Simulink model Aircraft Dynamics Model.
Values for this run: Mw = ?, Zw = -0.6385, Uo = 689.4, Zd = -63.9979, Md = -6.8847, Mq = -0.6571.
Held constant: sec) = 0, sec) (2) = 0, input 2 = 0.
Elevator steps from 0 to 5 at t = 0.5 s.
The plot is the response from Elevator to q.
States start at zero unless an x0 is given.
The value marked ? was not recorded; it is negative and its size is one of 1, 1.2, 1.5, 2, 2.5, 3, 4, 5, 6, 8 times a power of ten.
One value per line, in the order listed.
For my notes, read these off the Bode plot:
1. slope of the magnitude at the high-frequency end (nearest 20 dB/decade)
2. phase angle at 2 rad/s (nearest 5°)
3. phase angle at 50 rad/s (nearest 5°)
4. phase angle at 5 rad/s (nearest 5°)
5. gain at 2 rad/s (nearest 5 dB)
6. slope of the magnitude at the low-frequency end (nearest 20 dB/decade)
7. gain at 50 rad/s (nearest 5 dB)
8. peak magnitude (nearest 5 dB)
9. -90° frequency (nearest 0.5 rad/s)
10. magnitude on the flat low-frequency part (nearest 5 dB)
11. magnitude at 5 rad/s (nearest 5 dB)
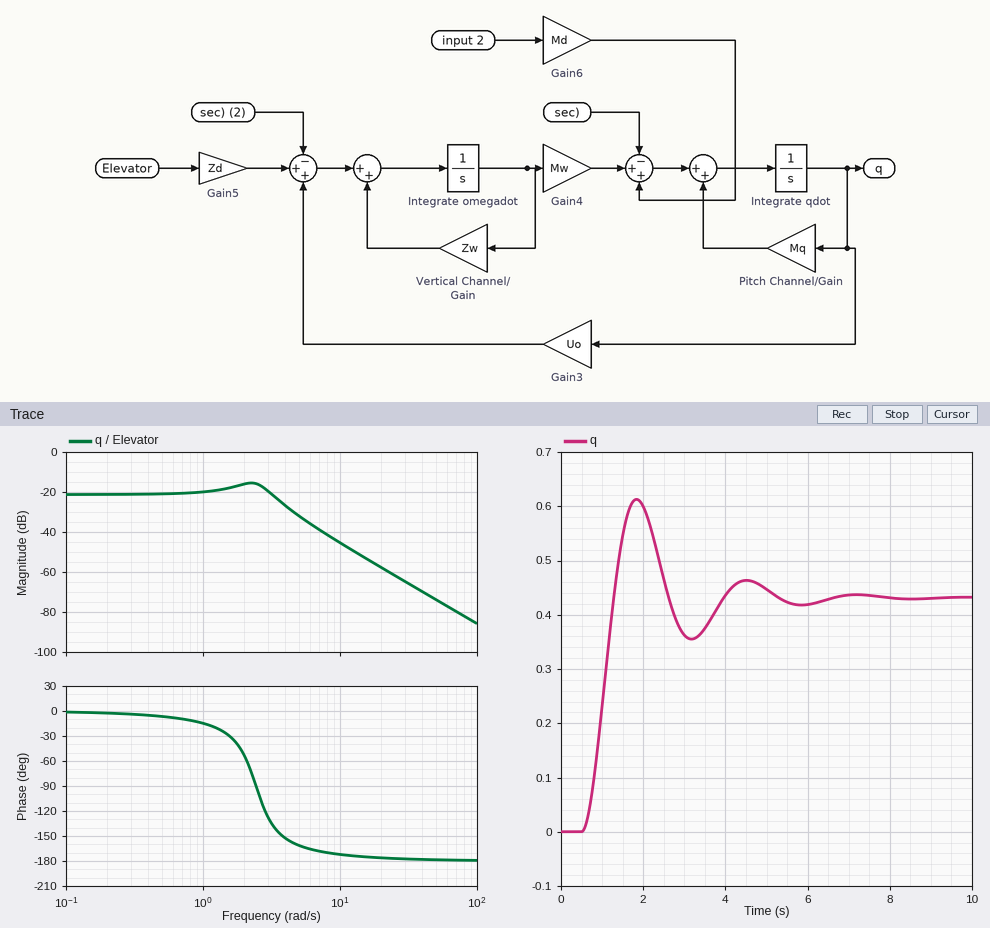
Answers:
-40 dB/decade
-55°
-180°
-160°
-15 dB
0 dB/decade
-75 dB
-15 dB
2.5 rad/s
-20 dB
-30 dB
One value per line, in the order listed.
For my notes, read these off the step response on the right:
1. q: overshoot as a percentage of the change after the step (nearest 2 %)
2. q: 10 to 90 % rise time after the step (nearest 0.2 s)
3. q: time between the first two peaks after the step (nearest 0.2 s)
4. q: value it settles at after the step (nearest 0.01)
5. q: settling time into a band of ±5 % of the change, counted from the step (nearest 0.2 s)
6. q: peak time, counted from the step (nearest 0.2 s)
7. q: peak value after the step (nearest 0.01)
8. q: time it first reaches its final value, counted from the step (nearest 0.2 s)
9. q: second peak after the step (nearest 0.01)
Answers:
42 %
0.6 s
2.6 s
0.43
4.4 s
1.4 s
0.61
0.8 s
0.46
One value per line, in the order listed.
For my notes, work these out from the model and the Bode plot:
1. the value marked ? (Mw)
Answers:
-0.008
